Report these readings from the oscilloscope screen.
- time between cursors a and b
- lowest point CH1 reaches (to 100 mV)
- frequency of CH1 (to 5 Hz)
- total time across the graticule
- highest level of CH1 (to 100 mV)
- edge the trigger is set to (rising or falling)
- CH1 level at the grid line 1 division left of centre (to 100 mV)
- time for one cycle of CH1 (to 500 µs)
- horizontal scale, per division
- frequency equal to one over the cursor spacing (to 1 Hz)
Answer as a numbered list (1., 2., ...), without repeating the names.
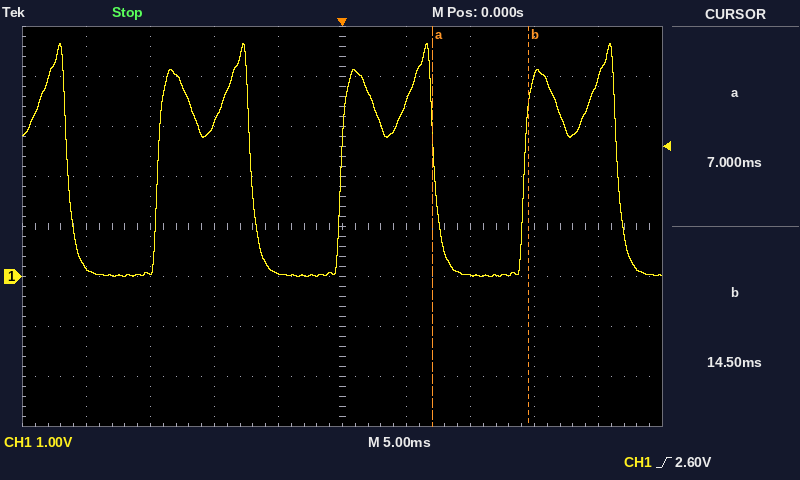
1. 7.5 ms
2. 0.0 V
3. 70 Hz
4. 50 ms
5. 4.7 V
6. rising
7. 100 mV
8. 14.5 ms
9. 5 ms
10. 133 Hz
